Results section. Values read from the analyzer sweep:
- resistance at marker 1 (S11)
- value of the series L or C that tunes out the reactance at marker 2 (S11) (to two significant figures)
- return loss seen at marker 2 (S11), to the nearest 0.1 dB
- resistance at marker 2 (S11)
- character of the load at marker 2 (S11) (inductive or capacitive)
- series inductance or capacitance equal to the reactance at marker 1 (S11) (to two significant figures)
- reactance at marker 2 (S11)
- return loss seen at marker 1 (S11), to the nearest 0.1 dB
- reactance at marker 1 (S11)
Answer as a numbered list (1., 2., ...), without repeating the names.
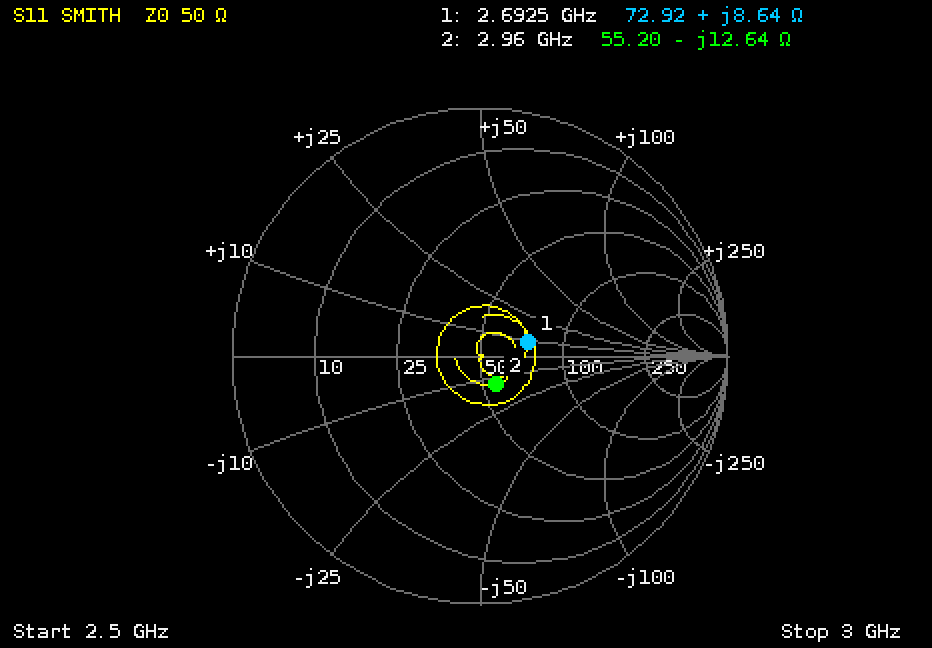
1. 72.92 Ω
2. 680 pH
3. 17.8 dB
4. 55.20 Ω
5. capacitive
6. 510 pH
7. -12.64 Ω
8. 14.0 dB
9. +8.64 Ω
